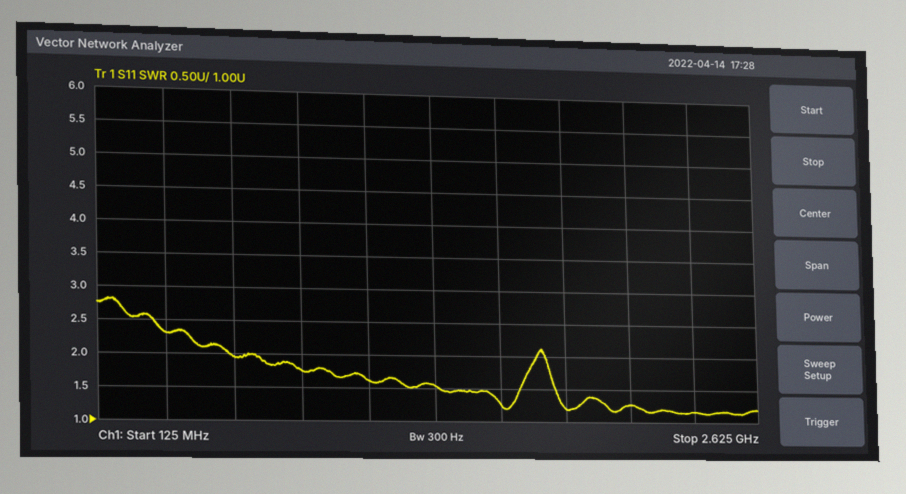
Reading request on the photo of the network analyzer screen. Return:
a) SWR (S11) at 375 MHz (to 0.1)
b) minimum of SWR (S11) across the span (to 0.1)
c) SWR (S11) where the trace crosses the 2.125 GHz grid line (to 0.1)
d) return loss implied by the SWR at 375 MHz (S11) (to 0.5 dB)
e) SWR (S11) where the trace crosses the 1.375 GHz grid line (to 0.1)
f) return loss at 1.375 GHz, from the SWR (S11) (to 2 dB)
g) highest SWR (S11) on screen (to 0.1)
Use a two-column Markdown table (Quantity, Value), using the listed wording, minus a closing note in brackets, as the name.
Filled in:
| Quantity | Value |
|---|---|
| SWR (S11) at 375 MHz | 2.3 |
| minimum of SWR (S11) across the span | 1.1 |
| SWR (S11) where the trace crosses the 2.125 GHz grid line | 1.3 |
| return loss implied by the SWR at 375 MHz (S11) | 8.0 dB |
| SWR (S11) where the trace crosses the 1.375 GHz grid line | 1.5 |
| return loss at 1.375 GHz, from the SWR (S11) | 14 dB |
| highest SWR (S11) on screen | 2.8 |
